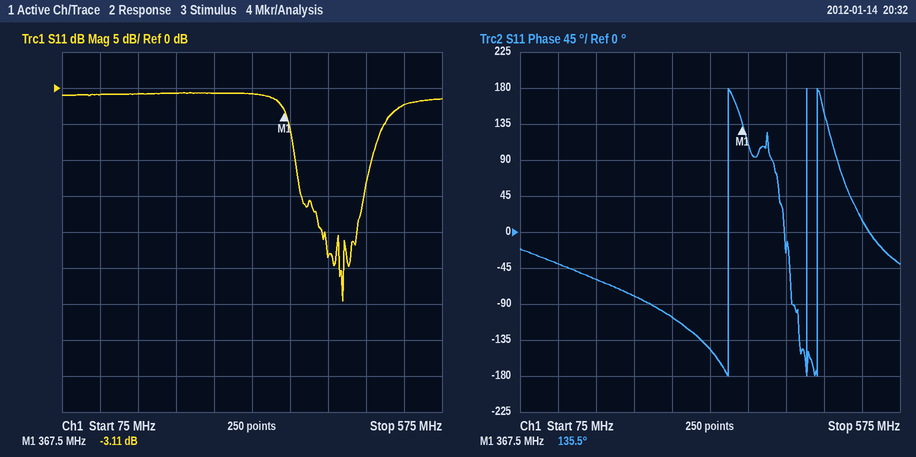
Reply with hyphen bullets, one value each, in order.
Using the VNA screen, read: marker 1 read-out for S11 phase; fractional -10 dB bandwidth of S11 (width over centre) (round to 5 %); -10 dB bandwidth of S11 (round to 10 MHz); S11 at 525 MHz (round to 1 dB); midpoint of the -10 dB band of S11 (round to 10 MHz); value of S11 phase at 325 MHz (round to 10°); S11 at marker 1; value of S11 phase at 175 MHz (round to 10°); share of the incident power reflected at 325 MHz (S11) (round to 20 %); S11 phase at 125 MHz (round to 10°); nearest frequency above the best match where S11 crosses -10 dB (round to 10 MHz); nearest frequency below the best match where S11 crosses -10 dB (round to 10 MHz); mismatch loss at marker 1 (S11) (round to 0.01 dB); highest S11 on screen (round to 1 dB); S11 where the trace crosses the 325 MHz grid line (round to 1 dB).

- 135.5°
- 25 %
- 100 MHz
- -2 dB
- 430 MHz
- -150°
- -3.11 dB
- -60°
- 80 %
- -40°
- 480 MHz
- 380 MHz
- 2.91 dB
- -1 dB
- -1 dB
